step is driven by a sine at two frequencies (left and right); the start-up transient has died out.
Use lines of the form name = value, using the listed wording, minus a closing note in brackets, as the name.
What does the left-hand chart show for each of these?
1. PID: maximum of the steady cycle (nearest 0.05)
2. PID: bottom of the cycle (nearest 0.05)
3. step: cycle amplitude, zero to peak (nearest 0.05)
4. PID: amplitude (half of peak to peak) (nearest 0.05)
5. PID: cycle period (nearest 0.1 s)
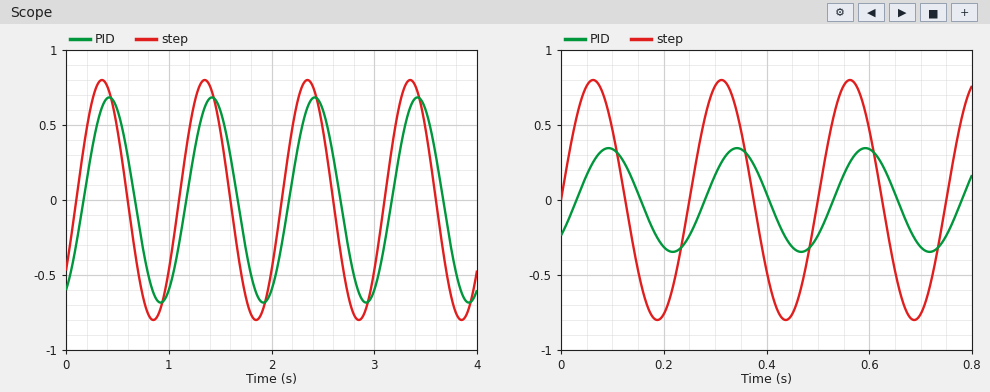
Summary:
PID: maximum of the steady cycle = 0.70
PID: bottom of the cycle = -0.70
step: cycle amplitude, zero to peak = 0.80
PID: amplitude (half of peak to peak) = 0.70
PID: cycle period = 1.0 s
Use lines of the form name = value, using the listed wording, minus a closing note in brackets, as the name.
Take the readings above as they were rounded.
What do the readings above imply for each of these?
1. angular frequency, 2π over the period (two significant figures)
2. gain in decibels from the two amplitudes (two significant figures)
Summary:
angular frequency, 2π over the period = 6.3 rad/s
gain in decibels from the two amplitudes = -1.2 dB
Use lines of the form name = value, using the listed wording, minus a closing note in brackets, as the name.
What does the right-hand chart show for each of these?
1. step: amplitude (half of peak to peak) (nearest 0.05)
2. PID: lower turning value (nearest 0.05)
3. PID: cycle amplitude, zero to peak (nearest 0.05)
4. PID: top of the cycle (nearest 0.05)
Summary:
step: amplitude (half of peak to peak) = 0.80
PID: lower turning value = -0.35
PID: cycle amplitude, zero to peak = 0.35
PID: top of the cycle = 0.35
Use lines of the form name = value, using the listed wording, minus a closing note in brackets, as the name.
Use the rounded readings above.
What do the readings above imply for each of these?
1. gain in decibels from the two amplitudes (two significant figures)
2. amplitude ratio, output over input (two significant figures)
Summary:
gain in decibels from the two amplitudes = -7.2 dB
amplitude ratio, output over input = 0.44
